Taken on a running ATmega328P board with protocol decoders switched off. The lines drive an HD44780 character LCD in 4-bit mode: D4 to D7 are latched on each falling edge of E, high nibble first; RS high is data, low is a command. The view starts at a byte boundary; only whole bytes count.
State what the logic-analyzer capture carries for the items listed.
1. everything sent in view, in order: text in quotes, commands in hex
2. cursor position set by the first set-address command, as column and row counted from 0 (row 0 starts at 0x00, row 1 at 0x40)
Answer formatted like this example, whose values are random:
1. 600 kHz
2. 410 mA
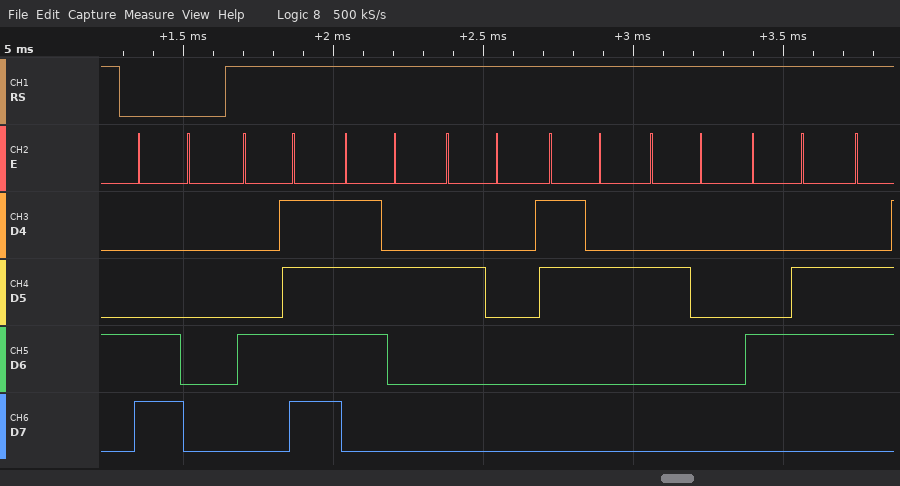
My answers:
1. 0xC0 "Or 2 F"
2. column 0, row 1
